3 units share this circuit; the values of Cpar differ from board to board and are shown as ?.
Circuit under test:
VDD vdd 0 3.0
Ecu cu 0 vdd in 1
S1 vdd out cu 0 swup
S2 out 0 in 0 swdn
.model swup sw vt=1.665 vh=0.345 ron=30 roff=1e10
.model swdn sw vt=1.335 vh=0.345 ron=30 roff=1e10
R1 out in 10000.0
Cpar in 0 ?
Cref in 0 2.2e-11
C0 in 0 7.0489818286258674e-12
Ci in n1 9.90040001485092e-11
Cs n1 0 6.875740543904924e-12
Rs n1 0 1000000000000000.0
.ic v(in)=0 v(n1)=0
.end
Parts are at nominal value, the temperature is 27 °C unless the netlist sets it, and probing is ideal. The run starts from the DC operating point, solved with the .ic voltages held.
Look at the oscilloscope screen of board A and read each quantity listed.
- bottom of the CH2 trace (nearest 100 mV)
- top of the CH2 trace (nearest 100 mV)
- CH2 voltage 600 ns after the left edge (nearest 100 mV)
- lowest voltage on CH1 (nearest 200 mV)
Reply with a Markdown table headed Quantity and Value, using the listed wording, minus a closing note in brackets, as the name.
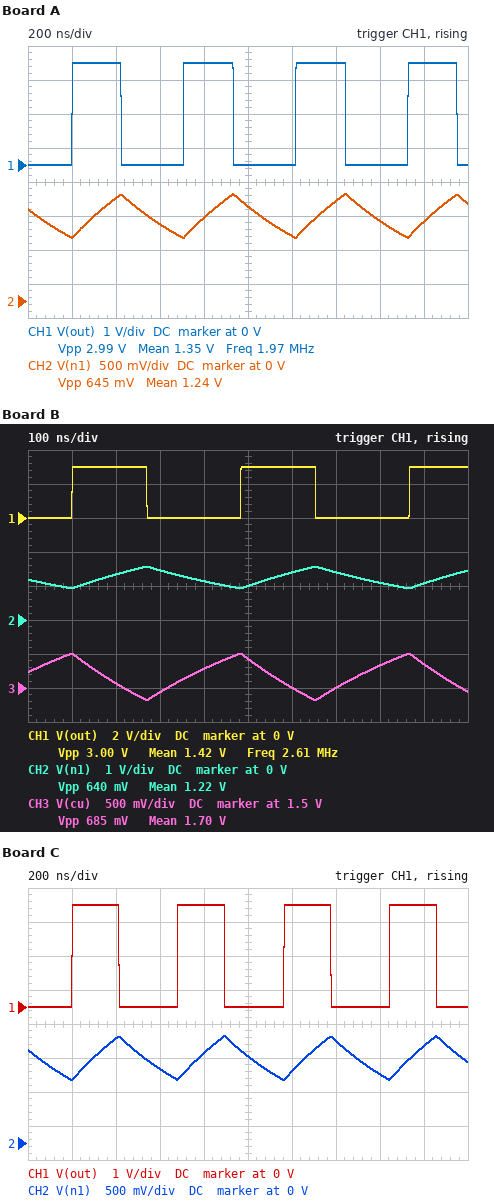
| Quantity | Value |
|---|---|
| bottom of the CH2 trace | 900 mV |
| top of the CH2 trace | 1.6 V |
| CH2 voltage 600 ns after the left edge | 1.1 V |
| lowest voltage on CH1 | 0 V |
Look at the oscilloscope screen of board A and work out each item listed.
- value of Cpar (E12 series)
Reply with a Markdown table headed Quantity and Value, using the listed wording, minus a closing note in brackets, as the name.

| Quantity | Value |
|---|---|
| value of Cpar | 18 pF |
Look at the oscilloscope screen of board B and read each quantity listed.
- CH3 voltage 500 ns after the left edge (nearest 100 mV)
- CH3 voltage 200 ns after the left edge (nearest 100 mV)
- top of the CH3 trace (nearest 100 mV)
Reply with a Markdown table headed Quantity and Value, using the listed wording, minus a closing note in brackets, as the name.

| Quantity | Value |
|---|---|
| CH3 voltage 500 ns after the left edge | 1.9 V |
| CH3 voltage 200 ns after the left edge | 1.6 V |
| top of the CH3 trace | 2.0 V |
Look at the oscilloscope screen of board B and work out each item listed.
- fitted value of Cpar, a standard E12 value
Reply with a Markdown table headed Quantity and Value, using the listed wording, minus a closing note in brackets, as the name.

| Quantity | Value |
|---|---|
| fitted value of Cpar, a standard E12 value | 4.7 pF |
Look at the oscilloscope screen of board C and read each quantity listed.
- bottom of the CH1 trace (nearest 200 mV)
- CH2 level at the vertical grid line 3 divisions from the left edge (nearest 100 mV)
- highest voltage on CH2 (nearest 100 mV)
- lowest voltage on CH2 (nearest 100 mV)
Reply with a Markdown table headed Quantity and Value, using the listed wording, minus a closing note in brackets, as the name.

| Quantity | Value |
|---|---|
| bottom of the CH1 trace | 0 V |
| CH2 level at the vertical grid line 3 divisions from the left edge | 1.1 V |
| highest voltage on CH2 | 1.6 V |
| lowest voltage on CH2 | 900 mV |
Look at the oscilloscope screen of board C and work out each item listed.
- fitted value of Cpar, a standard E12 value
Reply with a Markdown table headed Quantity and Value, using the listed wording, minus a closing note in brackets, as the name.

| Quantity | Value |
|---|---|
| fitted value of Cpar, a standard E12 value | 15 pF |
